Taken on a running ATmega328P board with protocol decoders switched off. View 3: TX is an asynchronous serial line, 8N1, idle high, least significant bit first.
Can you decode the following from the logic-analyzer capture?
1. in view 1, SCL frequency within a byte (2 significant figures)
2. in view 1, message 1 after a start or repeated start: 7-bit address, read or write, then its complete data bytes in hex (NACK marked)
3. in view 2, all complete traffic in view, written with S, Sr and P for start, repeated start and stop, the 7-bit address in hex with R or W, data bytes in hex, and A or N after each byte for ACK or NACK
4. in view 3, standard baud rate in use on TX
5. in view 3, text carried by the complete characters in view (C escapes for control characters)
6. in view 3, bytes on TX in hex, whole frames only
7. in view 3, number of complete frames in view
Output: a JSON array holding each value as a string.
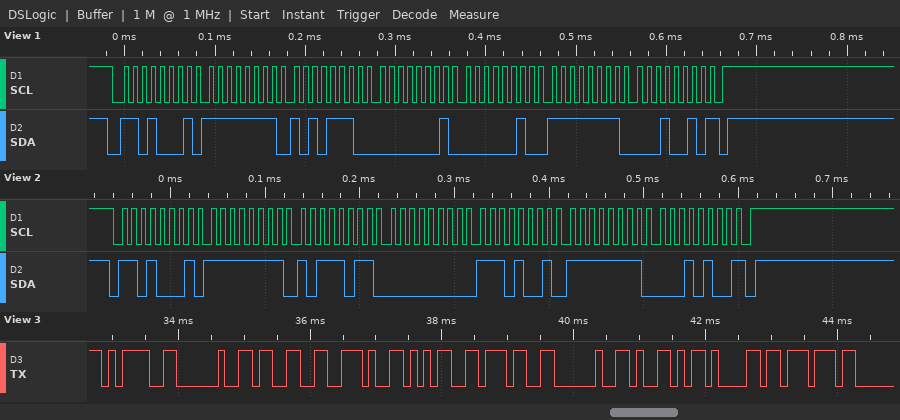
["100 kHz", "0x68 read: FF AE 01 02 FF 12 NACK", "S 68R A FF A BB A 00 A E9 A FF A 14 N P", "9600 baud", "\"= 3.57 Yaw\"", "3D 20 33 2E 35 37 20 59 61 77", "10"]
